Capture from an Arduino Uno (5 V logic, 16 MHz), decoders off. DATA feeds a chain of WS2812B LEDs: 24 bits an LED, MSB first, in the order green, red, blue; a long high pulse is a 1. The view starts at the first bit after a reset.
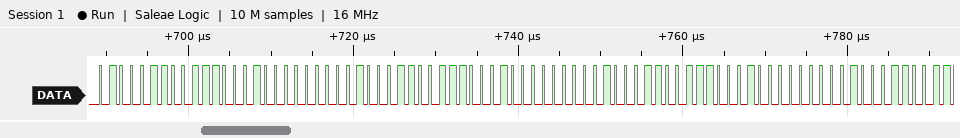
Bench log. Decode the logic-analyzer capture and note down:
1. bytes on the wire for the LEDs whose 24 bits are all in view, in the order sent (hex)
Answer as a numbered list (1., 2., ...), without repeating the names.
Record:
1. 46 71 00 46 71 00 46 71 00
